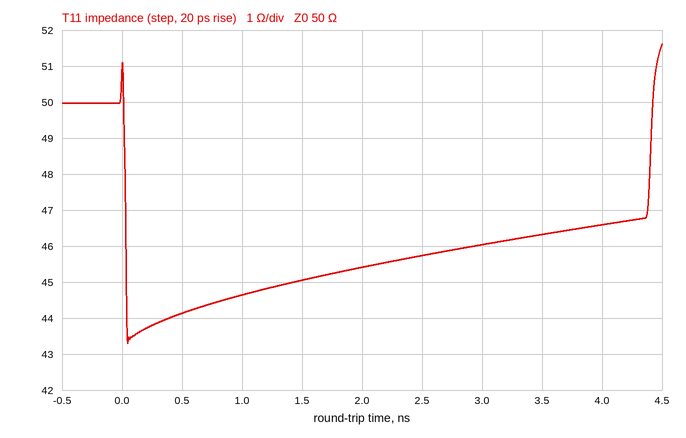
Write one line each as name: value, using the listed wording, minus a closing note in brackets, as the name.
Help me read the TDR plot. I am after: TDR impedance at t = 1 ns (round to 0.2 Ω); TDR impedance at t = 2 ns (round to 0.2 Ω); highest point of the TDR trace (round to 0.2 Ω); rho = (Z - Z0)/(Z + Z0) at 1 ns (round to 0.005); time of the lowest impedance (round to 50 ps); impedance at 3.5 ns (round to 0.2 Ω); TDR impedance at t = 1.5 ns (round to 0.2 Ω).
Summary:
TDR impedance at t = 1 ns: 44.6 Ω
TDR impedance at t = 2 ns: 45.4 Ω
highest point of the TDR trace: 51.6 Ω
rho = (Z - Z0)/(Z + Z0) at 1 ns: -0.055
time of the lowest impedance: 50 ps
impedance at 3.5 ns: 46.4 Ω
TDR impedance at t = 1.5 ns: 45.0 Ω
